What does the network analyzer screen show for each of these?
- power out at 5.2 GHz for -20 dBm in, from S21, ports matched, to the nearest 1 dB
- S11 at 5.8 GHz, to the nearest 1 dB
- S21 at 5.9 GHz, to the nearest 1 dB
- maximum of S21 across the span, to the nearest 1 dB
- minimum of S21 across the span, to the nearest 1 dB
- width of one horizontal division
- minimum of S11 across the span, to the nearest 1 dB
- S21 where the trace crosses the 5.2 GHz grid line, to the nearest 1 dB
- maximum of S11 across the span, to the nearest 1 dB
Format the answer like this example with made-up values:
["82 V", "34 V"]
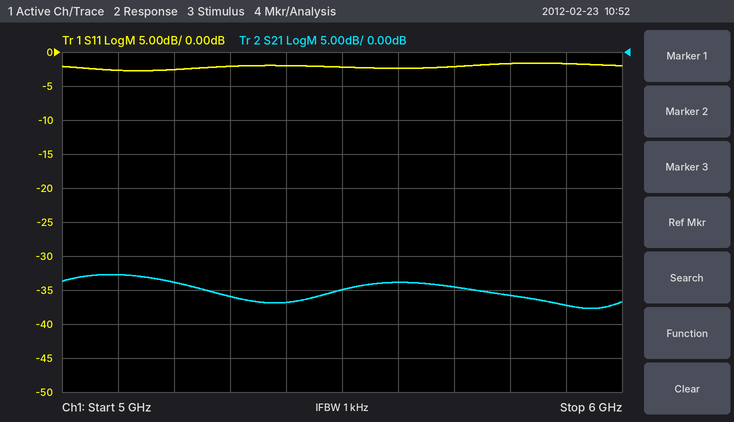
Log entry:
["-54 dBm", "-2 dB", "-37 dB", "-33 dB", "-38 dB", "100 MHz", "-3 dB", "-34 dB", "-2 dB"]
